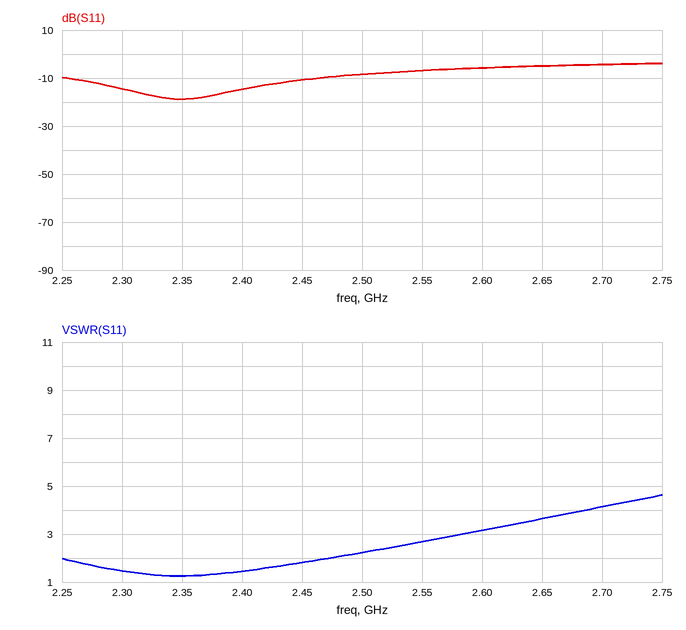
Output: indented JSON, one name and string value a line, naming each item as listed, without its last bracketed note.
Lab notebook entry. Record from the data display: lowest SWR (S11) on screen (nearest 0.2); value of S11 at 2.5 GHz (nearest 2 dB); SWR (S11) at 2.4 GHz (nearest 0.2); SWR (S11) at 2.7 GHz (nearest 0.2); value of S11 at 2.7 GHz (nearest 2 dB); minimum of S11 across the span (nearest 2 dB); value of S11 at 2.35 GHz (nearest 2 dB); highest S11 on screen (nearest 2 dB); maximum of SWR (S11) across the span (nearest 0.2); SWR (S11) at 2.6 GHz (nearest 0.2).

{
  "lowest SWR (S11) on screen": "1.2",
  "value of S11 at 2.5 GHz": "-8 dB",
  "SWR (S11) at 2.4 GHz": "1.4",
  "SWR (S11) at 2.7 GHz": "4.2",
  "value of S11 at 2.7 GHz": "-4 dB",
  "minimum of S11 across the span": "-18 dB",
  "value of S11 at 2.35 GHz": "-18 dB",
  "highest S11 on screen": "-4 dB",
  "maximum of SWR (S11) across the span": "4.6",
  "SWR (S11) at 2.6 GHz": "3.2"
}
